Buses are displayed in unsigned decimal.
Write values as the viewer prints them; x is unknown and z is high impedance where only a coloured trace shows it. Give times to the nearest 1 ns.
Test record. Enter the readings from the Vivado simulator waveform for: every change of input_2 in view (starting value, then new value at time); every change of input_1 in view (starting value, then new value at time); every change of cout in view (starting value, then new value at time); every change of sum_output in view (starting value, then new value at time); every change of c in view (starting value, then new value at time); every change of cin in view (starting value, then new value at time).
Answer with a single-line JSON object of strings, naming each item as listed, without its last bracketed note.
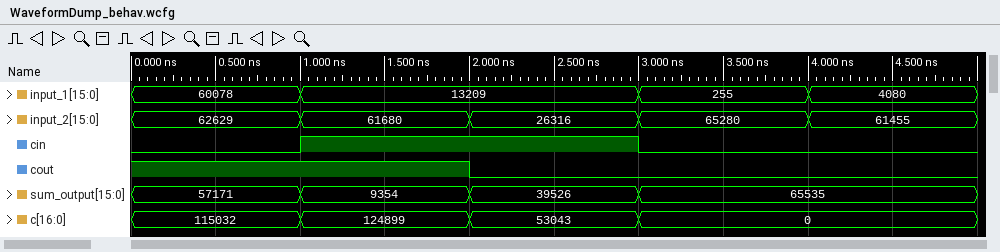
{"every change of input_2 in view": "62629, 61680 at 1 ns, 26316 at 2 ns, 65280 at 3 ns, 61455 at 4 ns", "every change of input_1 in view": "60078, 13209 at 1 ns, 255 at 3 ns, 4080 at 4 ns", "every change of cout in view": "1, 0 at 2 ns", "every change of sum_output in view": "57171, 9354 at 1 ns, 39526 at 2 ns, 65535 at 3 ns", "every change of c in view": "115032, 124899 at 1 ns, 53043 at 2 ns, 0 at 3 ns", "every change of cin in view": "0, 1 at 1 ns, 0 at 3 ns"}
